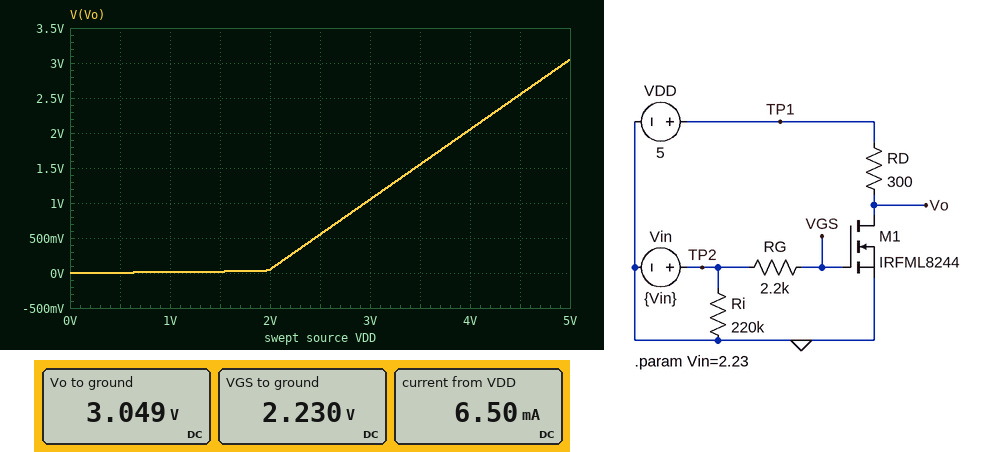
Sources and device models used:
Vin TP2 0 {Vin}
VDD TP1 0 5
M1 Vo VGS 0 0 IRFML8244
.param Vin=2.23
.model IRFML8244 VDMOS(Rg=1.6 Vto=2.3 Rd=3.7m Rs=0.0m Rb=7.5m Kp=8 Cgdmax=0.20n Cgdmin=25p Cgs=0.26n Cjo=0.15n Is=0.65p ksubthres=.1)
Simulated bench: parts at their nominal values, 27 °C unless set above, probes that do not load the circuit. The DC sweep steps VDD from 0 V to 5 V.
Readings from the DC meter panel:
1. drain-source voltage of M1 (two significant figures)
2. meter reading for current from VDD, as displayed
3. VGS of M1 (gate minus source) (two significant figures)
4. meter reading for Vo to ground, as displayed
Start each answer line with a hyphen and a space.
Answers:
- 3.0 V
- 6.50 mA
- 2.2 V
- 3.049 V
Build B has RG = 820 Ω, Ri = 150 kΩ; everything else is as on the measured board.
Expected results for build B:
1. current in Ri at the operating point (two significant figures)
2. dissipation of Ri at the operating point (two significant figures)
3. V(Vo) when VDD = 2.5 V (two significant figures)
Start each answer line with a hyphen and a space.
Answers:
- 15 µA
- 33 µW
- 550 mV
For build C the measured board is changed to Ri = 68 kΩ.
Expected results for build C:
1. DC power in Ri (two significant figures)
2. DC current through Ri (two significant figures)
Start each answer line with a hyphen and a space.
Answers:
- 73 µW
- 33 µA
